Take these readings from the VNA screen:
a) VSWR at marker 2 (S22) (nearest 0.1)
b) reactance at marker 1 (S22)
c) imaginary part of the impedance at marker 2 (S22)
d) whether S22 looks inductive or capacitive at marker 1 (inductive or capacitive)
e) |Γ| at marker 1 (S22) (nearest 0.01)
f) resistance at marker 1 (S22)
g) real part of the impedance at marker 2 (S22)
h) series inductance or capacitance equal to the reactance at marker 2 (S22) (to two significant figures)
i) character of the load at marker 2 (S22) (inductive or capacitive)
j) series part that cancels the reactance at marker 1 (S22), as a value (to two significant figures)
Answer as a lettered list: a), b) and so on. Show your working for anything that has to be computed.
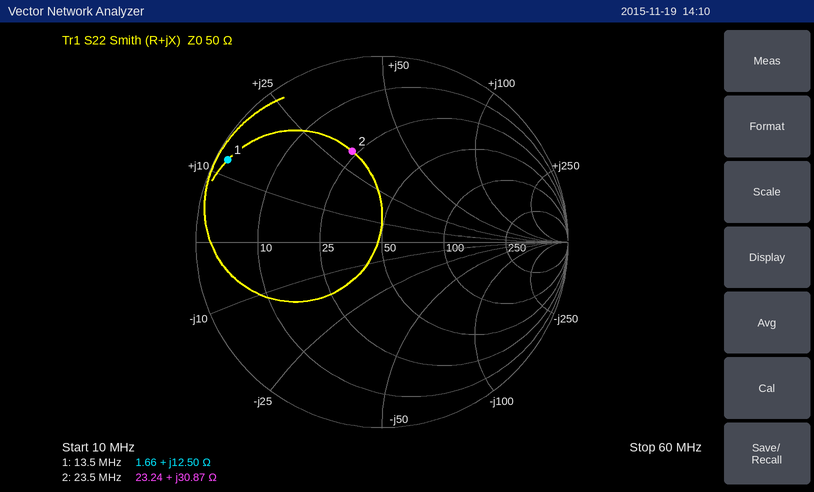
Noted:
a) 3.1
b) +12.50 Ω
c) +30.87 Ω
d) inductive
e) 0.94
f) 1.66 Ω
g) 23.24 Ω
h) L = 30.87 Ω/(2π × 23.5 MHz) ≈ 209 nH, so 210 nH to two significant figures
i) inductive
j) C = 1/(2π × 13.5 MHz × 12.5 Ω) ≈ 943 pF, so 940 pF to two significant figures
